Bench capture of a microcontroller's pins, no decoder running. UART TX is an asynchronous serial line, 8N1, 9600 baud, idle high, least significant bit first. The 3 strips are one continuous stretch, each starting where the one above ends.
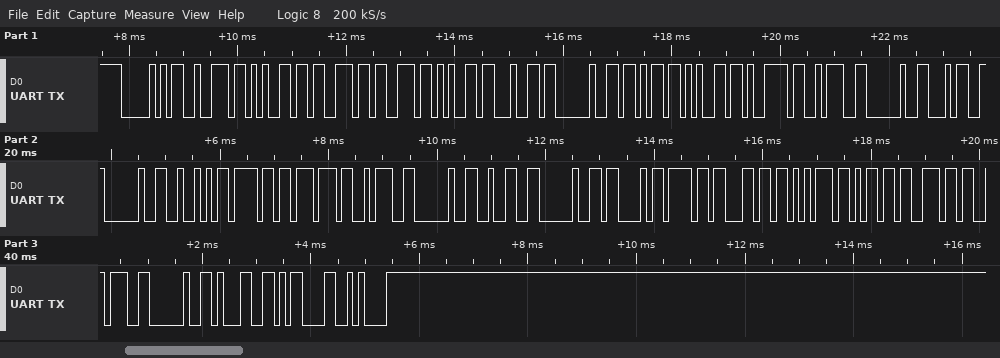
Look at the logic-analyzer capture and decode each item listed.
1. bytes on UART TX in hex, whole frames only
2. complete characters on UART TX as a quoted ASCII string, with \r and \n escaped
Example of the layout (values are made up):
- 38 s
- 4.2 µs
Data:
- 50 72 65 73 73 65 64 20 6B 65 79 3A 20 34 20 52 6F 77 3A 20 32 20 43 6F 6C 75 6D 6E 3A 20 31 0D 0A
- "Pressed key: 4 Row: 2 Column: 1\r\n"
